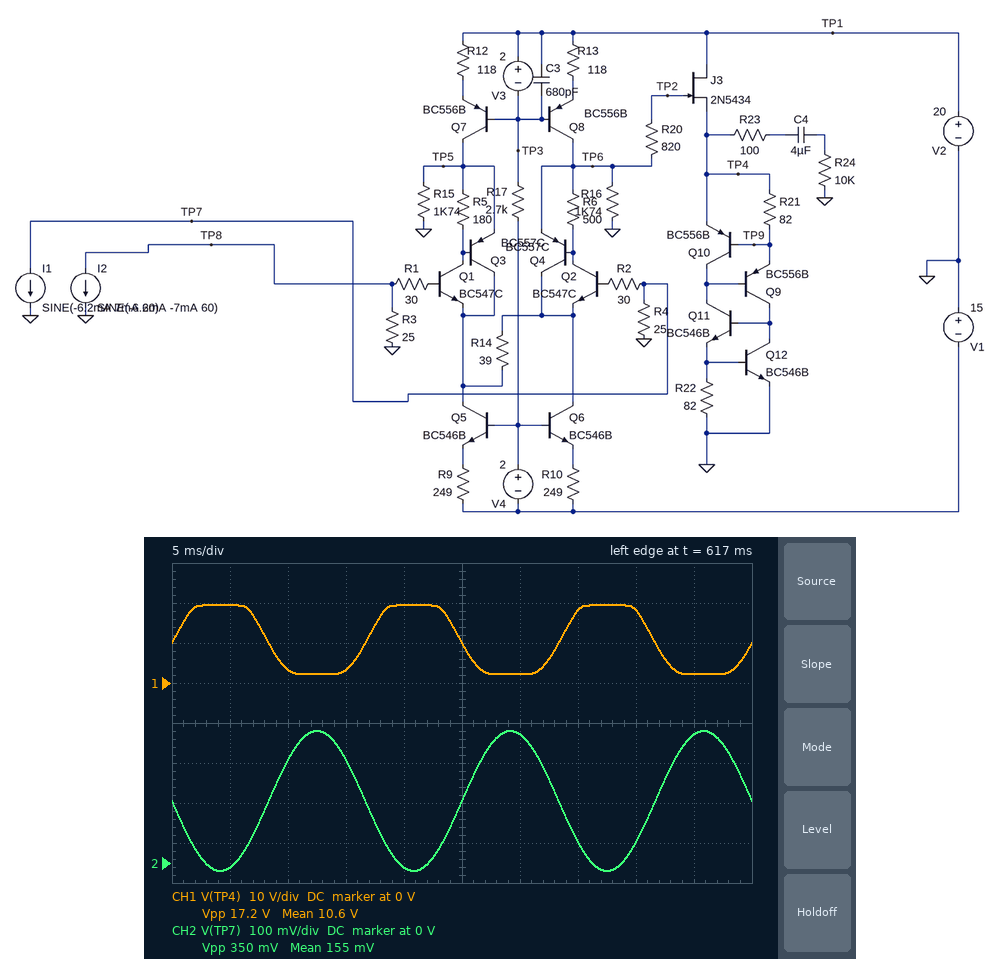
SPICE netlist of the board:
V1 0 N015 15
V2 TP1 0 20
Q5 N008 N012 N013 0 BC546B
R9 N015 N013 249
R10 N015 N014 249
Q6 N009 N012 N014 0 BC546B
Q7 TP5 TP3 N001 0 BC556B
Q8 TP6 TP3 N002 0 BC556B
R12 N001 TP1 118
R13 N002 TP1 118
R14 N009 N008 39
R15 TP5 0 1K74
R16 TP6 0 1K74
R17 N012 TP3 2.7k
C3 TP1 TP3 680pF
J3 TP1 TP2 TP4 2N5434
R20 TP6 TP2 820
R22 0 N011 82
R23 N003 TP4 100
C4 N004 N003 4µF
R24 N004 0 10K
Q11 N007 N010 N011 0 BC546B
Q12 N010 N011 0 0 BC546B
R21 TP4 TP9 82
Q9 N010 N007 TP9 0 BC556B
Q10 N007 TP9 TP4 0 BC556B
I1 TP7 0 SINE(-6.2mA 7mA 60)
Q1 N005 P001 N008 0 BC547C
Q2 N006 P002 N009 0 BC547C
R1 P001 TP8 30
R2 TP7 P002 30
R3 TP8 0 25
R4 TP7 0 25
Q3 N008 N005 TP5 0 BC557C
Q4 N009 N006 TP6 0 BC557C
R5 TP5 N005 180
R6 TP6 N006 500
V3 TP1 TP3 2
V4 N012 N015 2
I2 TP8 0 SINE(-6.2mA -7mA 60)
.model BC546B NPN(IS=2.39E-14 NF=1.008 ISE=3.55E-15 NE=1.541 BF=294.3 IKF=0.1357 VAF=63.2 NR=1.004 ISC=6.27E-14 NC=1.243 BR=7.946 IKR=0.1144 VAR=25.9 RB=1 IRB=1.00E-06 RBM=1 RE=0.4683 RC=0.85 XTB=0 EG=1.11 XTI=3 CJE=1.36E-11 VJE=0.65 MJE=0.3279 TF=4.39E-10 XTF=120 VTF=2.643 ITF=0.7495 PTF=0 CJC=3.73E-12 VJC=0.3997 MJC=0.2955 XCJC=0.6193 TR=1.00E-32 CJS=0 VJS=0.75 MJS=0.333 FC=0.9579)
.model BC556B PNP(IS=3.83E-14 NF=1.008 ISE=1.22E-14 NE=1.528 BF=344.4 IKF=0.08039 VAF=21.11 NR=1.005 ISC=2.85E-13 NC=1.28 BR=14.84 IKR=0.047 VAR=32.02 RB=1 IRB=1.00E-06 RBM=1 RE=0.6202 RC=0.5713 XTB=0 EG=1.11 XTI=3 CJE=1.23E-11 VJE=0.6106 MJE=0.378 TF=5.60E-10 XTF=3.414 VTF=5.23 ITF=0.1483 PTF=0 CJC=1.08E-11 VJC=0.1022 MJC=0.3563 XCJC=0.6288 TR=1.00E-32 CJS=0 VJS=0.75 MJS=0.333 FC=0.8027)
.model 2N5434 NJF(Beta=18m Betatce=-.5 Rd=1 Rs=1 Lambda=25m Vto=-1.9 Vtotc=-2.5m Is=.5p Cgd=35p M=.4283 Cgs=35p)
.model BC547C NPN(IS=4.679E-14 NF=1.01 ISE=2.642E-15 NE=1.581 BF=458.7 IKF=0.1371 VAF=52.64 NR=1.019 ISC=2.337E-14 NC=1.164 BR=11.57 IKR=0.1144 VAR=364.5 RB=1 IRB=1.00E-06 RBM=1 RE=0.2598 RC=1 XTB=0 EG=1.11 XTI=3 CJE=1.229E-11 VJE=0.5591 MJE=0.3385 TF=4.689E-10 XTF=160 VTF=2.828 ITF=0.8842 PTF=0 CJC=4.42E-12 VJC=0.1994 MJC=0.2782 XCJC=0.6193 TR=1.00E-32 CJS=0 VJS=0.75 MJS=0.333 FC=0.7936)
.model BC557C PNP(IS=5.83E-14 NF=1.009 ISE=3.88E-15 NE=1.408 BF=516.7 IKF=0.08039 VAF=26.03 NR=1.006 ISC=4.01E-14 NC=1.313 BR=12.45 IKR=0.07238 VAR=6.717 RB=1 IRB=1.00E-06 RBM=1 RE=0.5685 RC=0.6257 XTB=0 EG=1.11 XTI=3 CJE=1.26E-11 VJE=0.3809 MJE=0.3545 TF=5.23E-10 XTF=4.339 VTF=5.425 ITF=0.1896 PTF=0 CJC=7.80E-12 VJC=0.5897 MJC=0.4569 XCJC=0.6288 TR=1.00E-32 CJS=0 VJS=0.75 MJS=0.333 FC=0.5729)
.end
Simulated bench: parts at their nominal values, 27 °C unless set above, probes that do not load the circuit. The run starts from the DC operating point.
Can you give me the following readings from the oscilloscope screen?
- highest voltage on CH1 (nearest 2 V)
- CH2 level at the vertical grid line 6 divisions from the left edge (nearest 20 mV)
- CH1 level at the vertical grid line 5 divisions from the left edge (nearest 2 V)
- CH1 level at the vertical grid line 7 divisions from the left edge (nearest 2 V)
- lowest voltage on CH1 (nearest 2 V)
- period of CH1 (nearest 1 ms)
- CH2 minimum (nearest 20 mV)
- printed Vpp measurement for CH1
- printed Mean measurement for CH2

20 V
320 mV
10 V
18 V
2 V
17 ms
-20 mV
17.2 V
155 mV
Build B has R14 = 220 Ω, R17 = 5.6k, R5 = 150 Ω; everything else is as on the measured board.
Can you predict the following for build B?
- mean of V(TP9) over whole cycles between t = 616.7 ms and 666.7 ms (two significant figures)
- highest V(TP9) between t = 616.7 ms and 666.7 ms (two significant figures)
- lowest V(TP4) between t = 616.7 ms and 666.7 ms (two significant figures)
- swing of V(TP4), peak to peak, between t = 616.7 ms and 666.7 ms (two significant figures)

10 V
13 V
8.2 V
5.3 V
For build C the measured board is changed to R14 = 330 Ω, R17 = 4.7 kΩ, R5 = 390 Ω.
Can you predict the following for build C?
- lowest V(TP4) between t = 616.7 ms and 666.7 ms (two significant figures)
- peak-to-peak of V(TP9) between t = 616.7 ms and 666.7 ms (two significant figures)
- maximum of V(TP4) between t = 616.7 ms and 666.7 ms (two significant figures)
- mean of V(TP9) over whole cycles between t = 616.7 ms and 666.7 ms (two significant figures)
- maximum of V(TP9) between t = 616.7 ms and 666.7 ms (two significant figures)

9.3 V
3.6 V
13 V
10 V
12 V
